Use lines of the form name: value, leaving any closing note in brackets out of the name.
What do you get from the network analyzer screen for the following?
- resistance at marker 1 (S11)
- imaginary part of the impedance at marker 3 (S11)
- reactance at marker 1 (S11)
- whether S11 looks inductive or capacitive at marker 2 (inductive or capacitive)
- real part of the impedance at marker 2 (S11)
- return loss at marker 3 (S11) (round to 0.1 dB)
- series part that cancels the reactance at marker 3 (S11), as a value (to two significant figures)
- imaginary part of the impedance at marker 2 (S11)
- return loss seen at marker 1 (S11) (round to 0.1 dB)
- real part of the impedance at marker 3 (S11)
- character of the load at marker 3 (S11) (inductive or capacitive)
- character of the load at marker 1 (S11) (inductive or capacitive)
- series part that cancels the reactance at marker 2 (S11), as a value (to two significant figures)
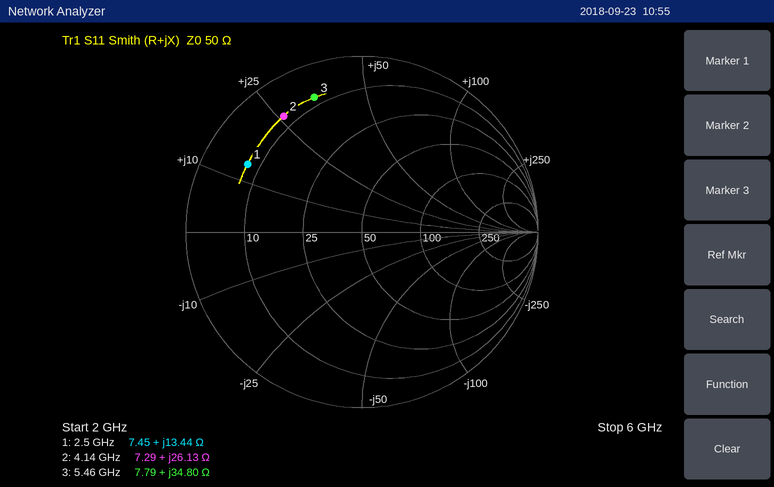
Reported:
resistance at marker 1: 7.45 Ω
imaginary part of the impedance at marker 3: +34.80 Ω
reactance at marker 1: +13.44 Ω
whether S11 looks inductive or capacitive at marker 2: inductive
real part of the impedance at marker 2: 7.29 Ω
return loss at marker 3 (S11): 1.8 dB
series part that cancels the reactance at marker 3 (S11), as a value: 840 fF
imaginary part of the impedance at marker 2: +26.13 Ω
return loss seen at marker 1 (S11): 2.4 dB
real part of the impedance at marker 3: 7.79 Ω
character of the load at marker 3 (S11): inductive
character of the load at marker 1 (S11): inductive
series part that cancels the reactance at marker 2 (S11), as a value: 1.5 pF
